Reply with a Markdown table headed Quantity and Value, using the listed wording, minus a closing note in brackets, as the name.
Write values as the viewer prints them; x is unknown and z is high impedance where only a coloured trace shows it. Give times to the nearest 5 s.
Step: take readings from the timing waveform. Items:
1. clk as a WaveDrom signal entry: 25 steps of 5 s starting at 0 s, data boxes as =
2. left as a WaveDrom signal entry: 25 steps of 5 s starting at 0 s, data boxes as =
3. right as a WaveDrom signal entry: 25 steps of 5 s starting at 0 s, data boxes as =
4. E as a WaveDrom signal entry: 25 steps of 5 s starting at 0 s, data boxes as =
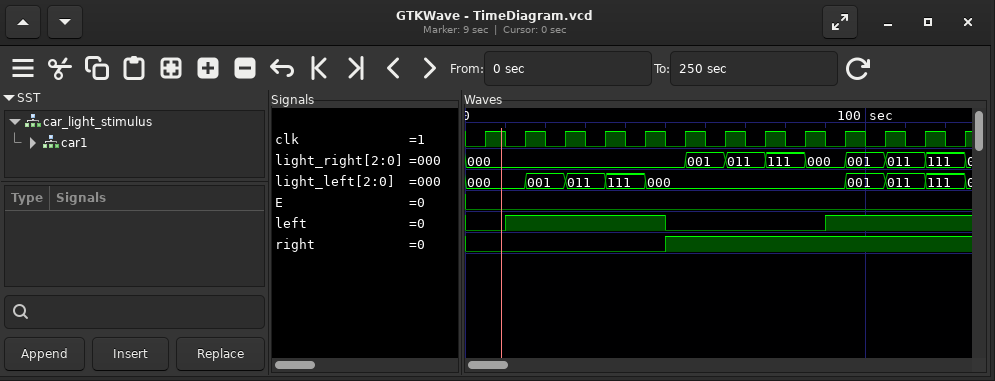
| Quantity | Value |
|---|---|
| clk as a WaveDrom signal entry: 25 steps of 5 s starting at 0 s, data boxes as = | {name: 'clk', wave: '0101010101010101010101010'} |
| left as a WaveDrom signal entry: 25 steps of 5 s starting at 0 s, data boxes as = | {name: 'left', wave: '0.1.......0.......1......'} |
| right as a WaveDrom signal entry: 25 steps of 5 s starting at 0 s, data boxes as = | {name: 'right', wave: '0.........1..............'} |
| E as a WaveDrom signal entry: 25 steps of 5 s starting at 0 s, data boxes as = | {name: 'E', wave: '0........................'} |
